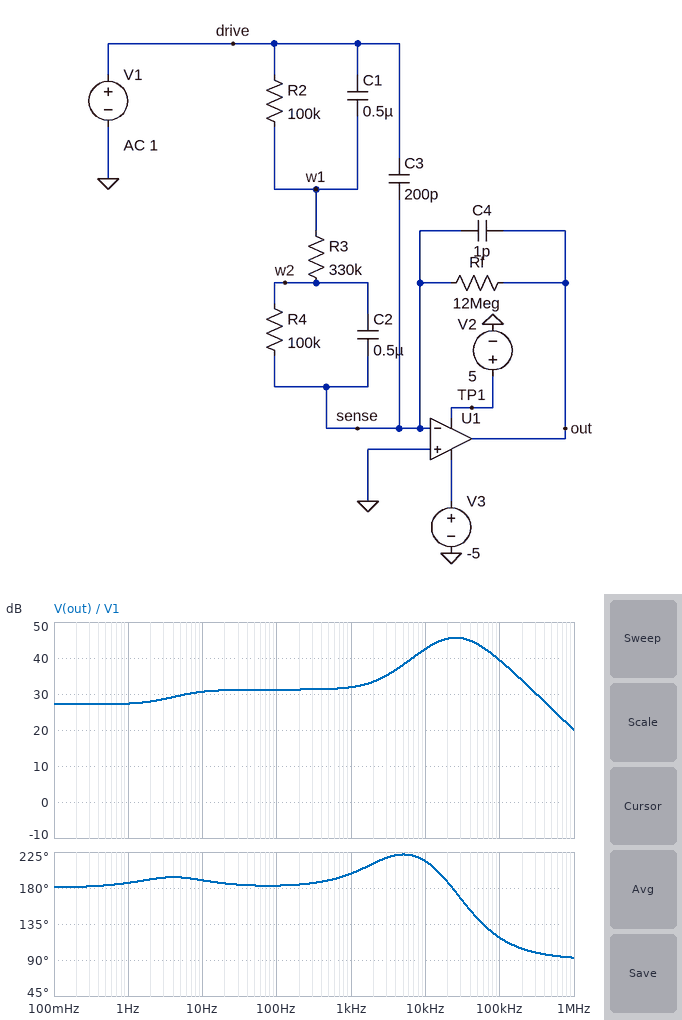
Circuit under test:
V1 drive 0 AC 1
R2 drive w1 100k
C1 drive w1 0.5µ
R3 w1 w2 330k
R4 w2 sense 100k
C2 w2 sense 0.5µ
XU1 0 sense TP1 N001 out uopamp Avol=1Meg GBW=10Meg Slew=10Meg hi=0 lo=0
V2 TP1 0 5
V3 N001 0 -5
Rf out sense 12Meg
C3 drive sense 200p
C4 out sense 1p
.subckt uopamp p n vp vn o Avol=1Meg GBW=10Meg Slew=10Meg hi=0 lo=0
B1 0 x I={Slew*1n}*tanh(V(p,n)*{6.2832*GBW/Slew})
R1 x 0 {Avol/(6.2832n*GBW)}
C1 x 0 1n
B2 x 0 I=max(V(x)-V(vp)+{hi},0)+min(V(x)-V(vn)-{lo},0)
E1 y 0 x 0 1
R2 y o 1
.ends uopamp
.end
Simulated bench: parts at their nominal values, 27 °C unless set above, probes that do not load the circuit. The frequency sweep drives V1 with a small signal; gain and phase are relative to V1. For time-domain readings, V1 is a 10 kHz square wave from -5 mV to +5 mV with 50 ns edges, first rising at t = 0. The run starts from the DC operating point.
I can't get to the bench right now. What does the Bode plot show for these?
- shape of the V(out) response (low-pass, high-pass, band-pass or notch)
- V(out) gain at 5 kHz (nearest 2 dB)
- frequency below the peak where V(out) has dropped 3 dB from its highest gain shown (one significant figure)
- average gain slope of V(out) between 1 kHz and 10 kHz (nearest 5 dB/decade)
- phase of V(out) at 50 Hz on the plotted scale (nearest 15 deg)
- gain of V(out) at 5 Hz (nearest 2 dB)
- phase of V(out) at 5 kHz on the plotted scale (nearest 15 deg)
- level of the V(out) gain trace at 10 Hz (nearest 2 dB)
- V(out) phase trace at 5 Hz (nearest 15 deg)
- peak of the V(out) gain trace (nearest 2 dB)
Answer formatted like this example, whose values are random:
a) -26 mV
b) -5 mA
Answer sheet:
a) band-pass
b) 38 dB
c) 10 kHz
d) 10 dB/decade
e) 180 deg
f) 30 dB
g) 225 deg
h) 30 dB
i) 195 deg
j) 46 dB
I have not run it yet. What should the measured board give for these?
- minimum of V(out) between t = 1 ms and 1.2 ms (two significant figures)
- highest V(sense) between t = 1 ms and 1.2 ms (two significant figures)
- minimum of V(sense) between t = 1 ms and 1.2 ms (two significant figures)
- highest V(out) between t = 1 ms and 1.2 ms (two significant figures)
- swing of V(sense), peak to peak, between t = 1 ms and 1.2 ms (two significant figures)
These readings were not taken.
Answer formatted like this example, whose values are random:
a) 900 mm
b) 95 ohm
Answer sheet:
a) -1.4 V
b) 9.9 mV
c) -9.9 mV
d) 1.3 V
e) 20 mV
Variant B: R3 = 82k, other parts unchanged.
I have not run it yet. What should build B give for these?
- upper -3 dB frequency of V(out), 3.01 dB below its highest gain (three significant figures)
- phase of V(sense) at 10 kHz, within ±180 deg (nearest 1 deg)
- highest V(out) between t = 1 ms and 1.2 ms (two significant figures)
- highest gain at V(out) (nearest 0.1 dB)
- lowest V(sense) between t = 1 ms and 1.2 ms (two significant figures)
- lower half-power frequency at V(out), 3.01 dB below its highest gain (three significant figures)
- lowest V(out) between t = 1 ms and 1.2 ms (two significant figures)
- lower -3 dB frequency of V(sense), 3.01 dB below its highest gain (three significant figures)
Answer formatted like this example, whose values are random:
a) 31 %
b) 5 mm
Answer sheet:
a) 61.8 kHz
b) 89 deg
c) 540 mV
d) 45.2 dB
e) -9.9 mV
f) 18.9 Hz
g) -1.5 V
h) 47.2 kHz
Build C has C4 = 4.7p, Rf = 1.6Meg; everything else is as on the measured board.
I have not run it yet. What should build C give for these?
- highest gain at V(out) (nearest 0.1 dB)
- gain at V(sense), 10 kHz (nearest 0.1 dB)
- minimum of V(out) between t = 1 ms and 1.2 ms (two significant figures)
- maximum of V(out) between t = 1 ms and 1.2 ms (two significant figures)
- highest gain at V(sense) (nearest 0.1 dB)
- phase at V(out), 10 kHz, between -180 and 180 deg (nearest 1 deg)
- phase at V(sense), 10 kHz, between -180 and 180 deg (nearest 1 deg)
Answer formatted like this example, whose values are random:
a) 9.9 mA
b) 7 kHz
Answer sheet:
a) 32.5 dB
b) -34.4 dB
c) -350 mV
d) 330 mV
e) -0.2 dB
f) -130 deg
g) 140 deg
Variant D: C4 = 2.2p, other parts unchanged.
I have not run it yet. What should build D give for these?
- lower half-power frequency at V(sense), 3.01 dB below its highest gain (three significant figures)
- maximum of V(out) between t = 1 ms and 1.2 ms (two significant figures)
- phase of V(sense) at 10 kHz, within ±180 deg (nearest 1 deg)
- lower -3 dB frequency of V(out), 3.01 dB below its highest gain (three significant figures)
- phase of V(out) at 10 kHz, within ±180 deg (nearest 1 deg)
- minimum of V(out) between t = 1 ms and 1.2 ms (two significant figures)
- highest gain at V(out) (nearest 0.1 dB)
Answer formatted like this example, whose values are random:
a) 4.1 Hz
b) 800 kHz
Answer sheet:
a) 105 kHz
b) 520 mV
c) 103 deg
d) 4.62 kHz
e) -167 deg
f) -660 mV
g) 39.0 dB
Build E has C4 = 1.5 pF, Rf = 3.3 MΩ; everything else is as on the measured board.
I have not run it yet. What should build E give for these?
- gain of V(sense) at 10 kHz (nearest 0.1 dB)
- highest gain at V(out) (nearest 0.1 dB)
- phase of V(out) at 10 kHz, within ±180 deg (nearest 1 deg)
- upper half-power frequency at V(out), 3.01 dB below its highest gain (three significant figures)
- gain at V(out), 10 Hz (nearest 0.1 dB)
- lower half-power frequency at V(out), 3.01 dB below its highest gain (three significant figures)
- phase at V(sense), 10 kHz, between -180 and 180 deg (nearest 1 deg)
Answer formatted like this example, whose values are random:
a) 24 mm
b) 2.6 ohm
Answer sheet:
a) -27.5 dB
b) 42.2 dB
c) -122 deg
d) 101 kHz
e) 19.4 dB
f) 23.6 kHz
g) 148 deg
